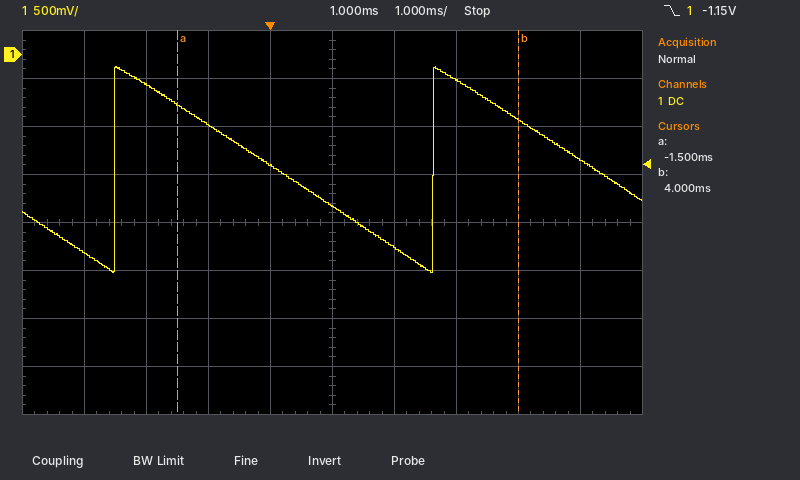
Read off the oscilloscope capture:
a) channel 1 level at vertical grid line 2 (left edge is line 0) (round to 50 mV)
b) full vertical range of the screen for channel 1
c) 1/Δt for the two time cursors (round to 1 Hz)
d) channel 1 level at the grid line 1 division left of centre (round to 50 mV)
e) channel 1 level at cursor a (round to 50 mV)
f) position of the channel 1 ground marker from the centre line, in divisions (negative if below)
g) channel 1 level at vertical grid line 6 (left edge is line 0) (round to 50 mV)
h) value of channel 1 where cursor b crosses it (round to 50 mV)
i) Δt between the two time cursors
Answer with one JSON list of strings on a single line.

["-300 mV", "4 V", "182 Hz", "-1.15 V", "-500 mV", "+3.5 div", "-2.00 V", "-700 mV", "5.5 ms"]
